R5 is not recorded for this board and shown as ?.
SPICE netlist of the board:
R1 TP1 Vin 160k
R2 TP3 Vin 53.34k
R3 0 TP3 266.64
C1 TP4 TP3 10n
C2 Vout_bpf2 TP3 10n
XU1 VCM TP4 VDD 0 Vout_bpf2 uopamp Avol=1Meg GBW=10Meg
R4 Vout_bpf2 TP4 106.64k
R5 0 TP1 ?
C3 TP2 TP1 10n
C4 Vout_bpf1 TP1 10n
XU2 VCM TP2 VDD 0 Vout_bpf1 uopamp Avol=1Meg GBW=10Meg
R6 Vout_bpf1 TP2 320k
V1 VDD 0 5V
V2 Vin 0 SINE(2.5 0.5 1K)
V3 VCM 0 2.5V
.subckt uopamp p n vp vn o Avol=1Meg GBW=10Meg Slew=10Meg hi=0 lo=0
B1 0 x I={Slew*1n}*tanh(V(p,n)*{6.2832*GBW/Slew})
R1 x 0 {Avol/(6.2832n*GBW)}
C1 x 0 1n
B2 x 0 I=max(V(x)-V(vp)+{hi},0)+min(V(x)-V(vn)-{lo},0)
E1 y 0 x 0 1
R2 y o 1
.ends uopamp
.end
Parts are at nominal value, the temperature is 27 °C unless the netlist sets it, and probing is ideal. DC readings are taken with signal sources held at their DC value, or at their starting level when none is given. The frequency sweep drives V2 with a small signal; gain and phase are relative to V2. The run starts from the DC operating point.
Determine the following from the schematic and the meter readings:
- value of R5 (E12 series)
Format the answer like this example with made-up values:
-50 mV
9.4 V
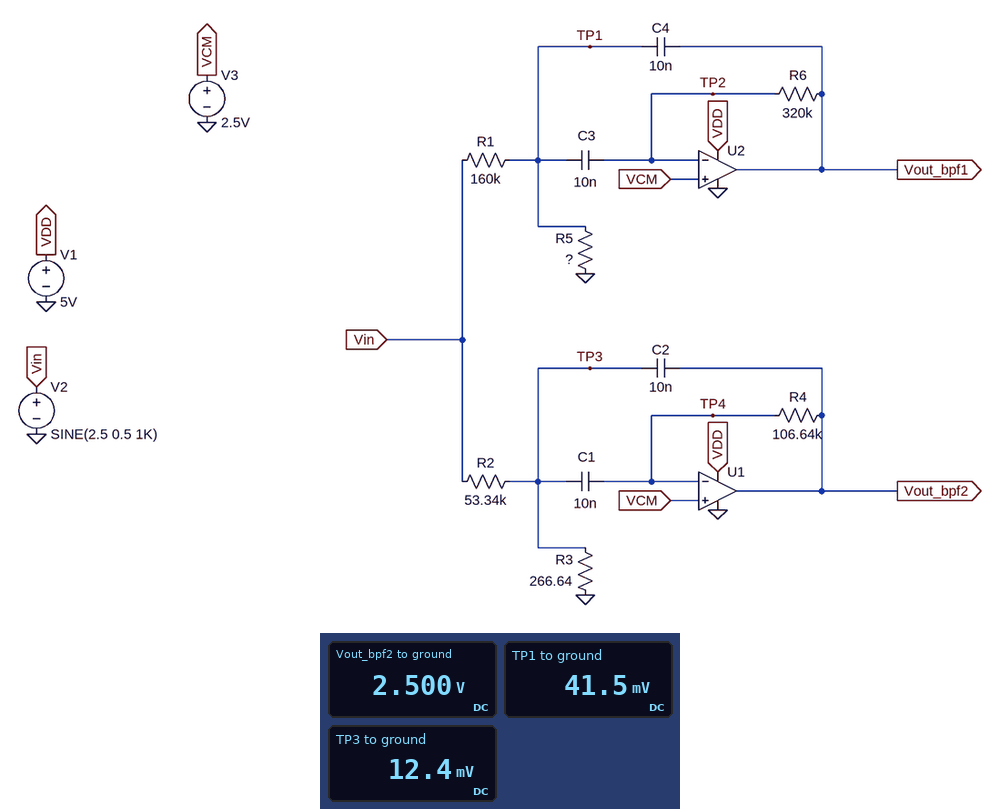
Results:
2.7 kΩ
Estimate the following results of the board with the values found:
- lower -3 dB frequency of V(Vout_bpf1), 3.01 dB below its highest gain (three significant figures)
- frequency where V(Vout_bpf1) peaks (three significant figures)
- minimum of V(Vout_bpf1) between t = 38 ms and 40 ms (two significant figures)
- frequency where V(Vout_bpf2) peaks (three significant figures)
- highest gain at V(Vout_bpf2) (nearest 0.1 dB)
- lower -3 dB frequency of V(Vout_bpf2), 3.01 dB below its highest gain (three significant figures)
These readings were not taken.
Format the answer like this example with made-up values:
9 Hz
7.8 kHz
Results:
498 Hz
546 Hz
2.4 V
2.98 kHz
0 dB
2.84 kHz
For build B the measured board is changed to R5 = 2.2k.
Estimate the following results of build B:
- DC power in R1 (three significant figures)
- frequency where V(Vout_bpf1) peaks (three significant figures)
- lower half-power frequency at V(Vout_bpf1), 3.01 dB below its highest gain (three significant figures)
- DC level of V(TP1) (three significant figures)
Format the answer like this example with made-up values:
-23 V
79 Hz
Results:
38.0 µW
604 Hz
556 Hz
33.9 mV
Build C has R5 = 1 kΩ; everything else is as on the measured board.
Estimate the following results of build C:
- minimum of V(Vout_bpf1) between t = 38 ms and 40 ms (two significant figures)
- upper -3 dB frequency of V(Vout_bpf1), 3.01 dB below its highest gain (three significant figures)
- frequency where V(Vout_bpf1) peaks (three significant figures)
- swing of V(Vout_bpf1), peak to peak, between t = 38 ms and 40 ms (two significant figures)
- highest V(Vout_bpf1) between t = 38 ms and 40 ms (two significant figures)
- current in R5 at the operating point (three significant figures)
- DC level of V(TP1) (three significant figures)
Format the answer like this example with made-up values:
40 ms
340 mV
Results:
2.3 V
943 Hz
892 Hz
440 mV
2.7 V
15.5 µA
15.5 mV
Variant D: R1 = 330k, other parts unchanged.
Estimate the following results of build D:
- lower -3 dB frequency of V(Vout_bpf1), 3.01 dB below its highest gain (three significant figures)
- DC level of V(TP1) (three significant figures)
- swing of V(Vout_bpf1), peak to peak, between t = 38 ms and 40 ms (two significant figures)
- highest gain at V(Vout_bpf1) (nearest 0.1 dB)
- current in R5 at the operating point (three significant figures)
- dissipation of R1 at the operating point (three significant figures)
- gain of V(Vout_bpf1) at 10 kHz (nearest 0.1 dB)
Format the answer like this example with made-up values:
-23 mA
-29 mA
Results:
496 Hz
20.3 mV
68 mV
-6.3 dB
7.51 µA
18.6 µW
-46.3 dB
